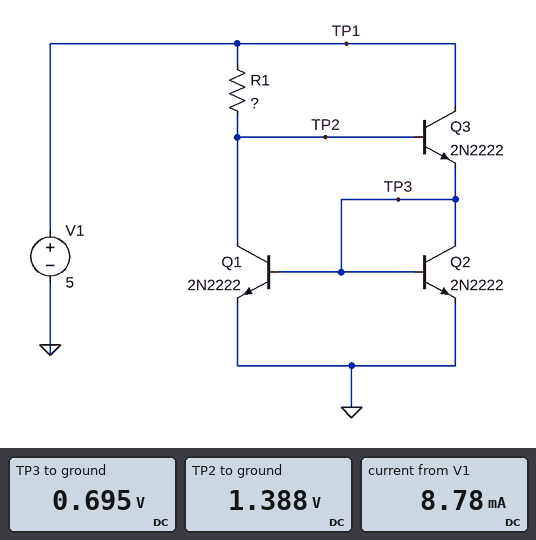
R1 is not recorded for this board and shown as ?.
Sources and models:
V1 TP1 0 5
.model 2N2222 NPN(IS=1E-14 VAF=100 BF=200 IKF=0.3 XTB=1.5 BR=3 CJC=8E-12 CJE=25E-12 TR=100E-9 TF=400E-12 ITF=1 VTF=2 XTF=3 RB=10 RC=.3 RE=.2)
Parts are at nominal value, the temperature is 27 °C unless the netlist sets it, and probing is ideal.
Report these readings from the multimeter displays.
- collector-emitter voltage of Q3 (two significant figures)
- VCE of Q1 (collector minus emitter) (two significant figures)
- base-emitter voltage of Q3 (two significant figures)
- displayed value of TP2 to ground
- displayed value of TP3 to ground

4.3 V
1.4 V
690 mV
1.388 V
0.695 V
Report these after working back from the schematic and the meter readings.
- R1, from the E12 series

820 Ω
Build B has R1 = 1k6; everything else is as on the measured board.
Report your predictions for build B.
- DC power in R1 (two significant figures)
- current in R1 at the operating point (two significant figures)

8.3 mW
2.3 mA
